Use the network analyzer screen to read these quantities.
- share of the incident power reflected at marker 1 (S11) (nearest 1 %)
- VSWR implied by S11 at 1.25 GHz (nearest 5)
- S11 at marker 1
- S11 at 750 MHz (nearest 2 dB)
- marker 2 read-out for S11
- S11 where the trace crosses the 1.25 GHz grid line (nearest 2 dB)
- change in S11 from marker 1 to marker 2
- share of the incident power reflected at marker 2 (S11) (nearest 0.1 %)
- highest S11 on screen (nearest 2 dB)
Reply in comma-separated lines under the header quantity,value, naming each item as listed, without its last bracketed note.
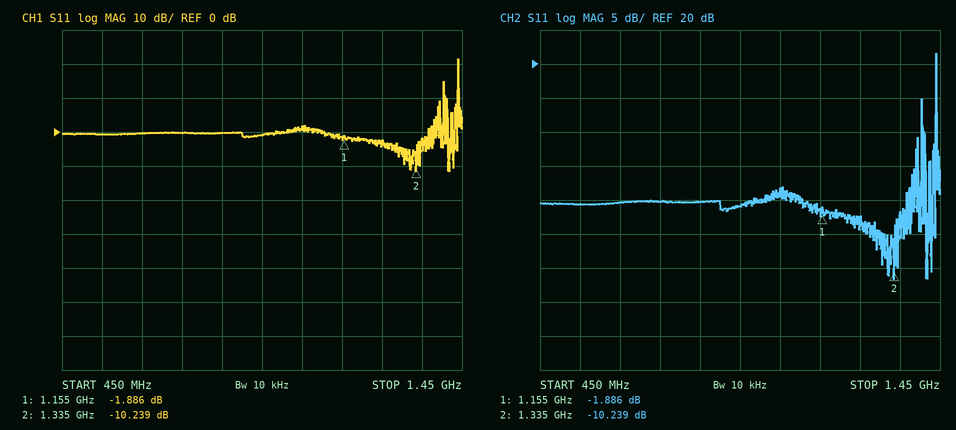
quantity,value
share of the incident power reflected at marker 1 (S11),65 %
VSWR implied by S11 at 1.25 GHz,5
S11 at marker 1,-1.886 dB
S11 at 750 MHz,0 dB
marker 2 read-out for S11,-10.239 dB
S11 where the trace crosses the 1.25 GHz grid line,-4 dB
change in S11 from marker 1 to marker 2,-8.353 dB
share of the incident power reflected at marker 2 (S11),9.5 %
highest S11 on screen,22 dB
